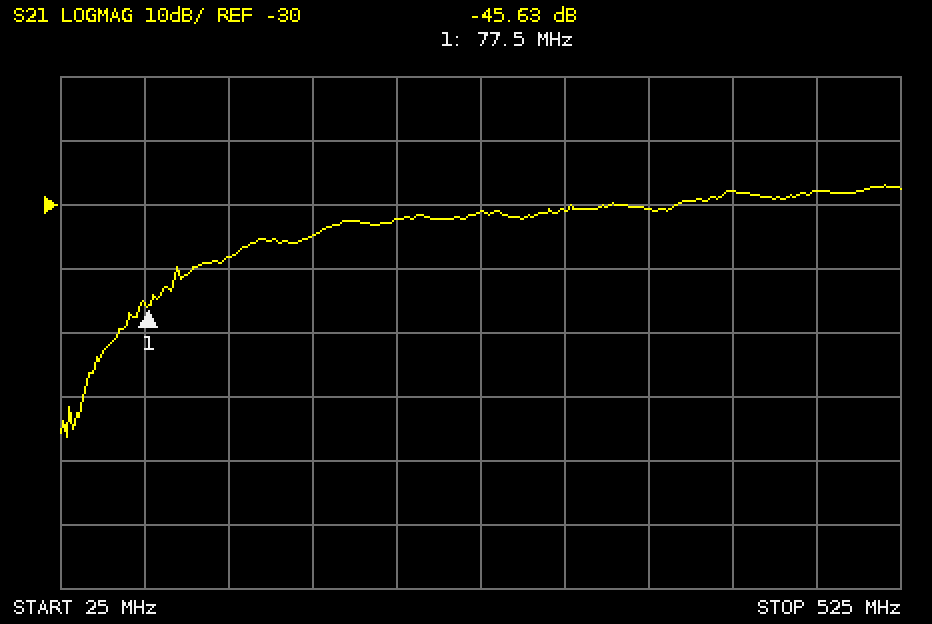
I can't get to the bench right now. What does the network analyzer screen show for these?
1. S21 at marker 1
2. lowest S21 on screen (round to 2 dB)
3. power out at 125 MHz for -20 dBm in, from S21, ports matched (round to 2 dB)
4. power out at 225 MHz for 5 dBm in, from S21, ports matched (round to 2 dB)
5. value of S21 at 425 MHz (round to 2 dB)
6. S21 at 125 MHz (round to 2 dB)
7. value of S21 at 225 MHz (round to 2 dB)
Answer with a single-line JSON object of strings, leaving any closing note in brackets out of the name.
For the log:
{"S21 at marker 1": "-45.63 dB", "lowest S21 on screen": "-66 dB", "power out at 125 MHz for -20 dBm in, from S21, ports matched": "-58 dBm", "power out at 225 MHz for 5 dBm in, from S21, ports matched": "-28 dBm", "value of S21 at 425 MHz": "-28 dB", "S21 at 125 MHz": "-38 dB", "value of S21 at 225 MHz": "-32 dB"}
